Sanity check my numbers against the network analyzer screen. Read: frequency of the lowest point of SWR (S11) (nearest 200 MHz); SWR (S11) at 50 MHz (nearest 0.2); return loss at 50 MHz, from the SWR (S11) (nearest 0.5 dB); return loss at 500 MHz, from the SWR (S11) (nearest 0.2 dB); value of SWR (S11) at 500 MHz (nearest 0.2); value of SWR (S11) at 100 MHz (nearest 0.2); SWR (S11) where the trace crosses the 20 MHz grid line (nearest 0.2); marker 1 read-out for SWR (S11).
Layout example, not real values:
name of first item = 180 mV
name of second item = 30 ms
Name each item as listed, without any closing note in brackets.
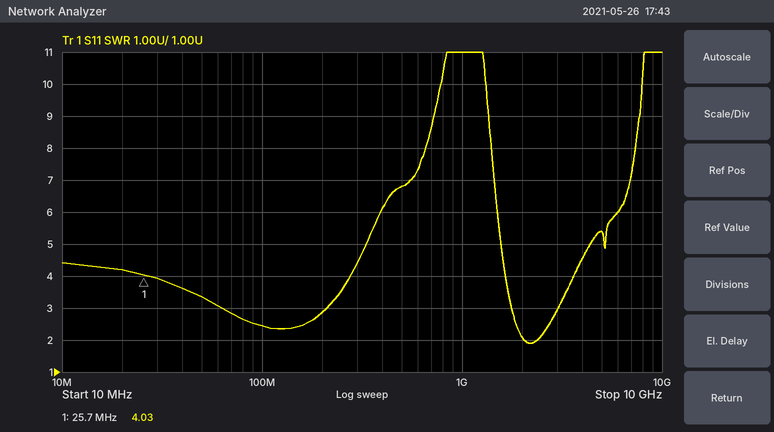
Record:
frequency of the lowest point of SWR (S11) = 2.2 GHz
SWR (S11) at 50 MHz = 3.4
return loss at 50 MHz, from the SWR (S11) = 5.5 dB
return loss at 500 MHz, from the SWR (S11) = 2.6 dB
value of SWR (S11) at 500 MHz = 6.8
value of SWR (S11) at 100 MHz = 2.4
SWR (S11) where the trace crosses the 20 MHz grid line = 4.2
marker 1 read-out for SWR = 4.03
